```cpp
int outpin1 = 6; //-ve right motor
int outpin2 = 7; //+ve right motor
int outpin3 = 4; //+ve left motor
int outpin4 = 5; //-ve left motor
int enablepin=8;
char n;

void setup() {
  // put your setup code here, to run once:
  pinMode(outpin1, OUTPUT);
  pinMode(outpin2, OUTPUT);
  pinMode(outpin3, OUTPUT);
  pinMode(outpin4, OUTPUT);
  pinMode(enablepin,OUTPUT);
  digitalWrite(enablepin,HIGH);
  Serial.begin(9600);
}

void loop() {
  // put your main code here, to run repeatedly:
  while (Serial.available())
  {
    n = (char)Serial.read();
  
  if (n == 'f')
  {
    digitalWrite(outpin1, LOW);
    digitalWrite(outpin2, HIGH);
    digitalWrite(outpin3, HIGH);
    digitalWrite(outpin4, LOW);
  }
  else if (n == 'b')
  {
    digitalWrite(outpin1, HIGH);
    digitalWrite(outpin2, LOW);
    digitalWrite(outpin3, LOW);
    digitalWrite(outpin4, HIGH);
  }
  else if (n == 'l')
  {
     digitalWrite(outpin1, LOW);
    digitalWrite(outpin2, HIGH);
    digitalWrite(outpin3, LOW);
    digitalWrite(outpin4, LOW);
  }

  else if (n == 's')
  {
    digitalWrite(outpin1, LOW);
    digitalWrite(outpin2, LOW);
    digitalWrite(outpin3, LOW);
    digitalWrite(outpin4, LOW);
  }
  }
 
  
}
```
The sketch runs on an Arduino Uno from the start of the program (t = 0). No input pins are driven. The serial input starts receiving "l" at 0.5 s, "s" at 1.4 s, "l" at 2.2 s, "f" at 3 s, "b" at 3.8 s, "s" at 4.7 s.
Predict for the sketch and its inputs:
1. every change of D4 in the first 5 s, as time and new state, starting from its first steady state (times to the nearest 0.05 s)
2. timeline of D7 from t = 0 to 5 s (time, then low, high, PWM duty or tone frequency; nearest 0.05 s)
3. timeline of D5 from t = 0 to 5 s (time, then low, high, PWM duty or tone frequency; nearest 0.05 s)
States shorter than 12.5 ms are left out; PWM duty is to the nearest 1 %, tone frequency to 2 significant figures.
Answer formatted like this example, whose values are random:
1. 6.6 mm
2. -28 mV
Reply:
1. 0 s low; 3 s high; 3.8 s low
2. 0 s low; 0.5 s high; 1.4 s low; 2.2 s high; 3.8 s low
3. 0 s low; 3.8 s high; 4.7 s low
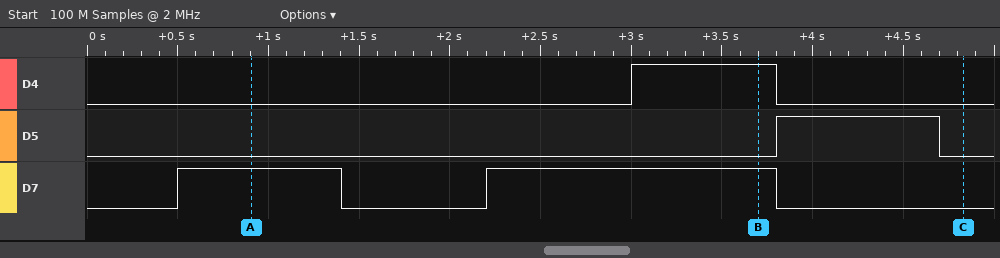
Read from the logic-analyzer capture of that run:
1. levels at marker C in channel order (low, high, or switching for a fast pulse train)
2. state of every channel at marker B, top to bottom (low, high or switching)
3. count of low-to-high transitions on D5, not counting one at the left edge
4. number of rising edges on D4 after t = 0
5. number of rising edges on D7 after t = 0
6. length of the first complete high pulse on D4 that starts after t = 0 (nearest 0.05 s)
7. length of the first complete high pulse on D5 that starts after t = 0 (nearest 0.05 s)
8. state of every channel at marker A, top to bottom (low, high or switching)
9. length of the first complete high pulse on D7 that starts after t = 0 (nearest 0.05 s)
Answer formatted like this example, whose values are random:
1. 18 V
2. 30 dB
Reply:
1. D4 low, D5 low, D7 low
2. D4 high, D5 low, D7 high
3. 1
4. 1
5. 2
6. 0.80 s
7. 0.90 s
8. D4 low, D5 low, D7 high
9. 0.90 s
